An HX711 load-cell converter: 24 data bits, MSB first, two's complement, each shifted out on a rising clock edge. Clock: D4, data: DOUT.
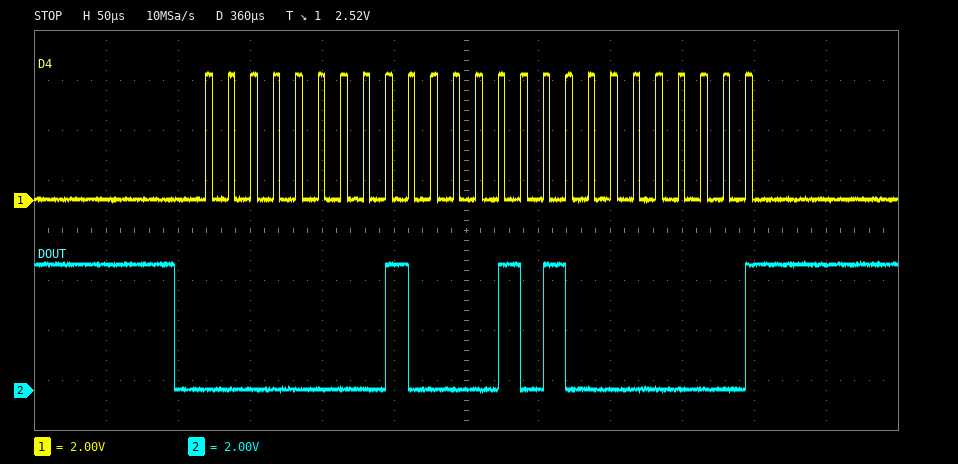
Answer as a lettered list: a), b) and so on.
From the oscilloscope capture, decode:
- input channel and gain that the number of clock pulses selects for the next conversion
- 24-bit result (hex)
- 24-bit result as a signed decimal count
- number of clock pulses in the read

a) channel A, gain 128
b) 0x008500
c) 34048
d) 25
